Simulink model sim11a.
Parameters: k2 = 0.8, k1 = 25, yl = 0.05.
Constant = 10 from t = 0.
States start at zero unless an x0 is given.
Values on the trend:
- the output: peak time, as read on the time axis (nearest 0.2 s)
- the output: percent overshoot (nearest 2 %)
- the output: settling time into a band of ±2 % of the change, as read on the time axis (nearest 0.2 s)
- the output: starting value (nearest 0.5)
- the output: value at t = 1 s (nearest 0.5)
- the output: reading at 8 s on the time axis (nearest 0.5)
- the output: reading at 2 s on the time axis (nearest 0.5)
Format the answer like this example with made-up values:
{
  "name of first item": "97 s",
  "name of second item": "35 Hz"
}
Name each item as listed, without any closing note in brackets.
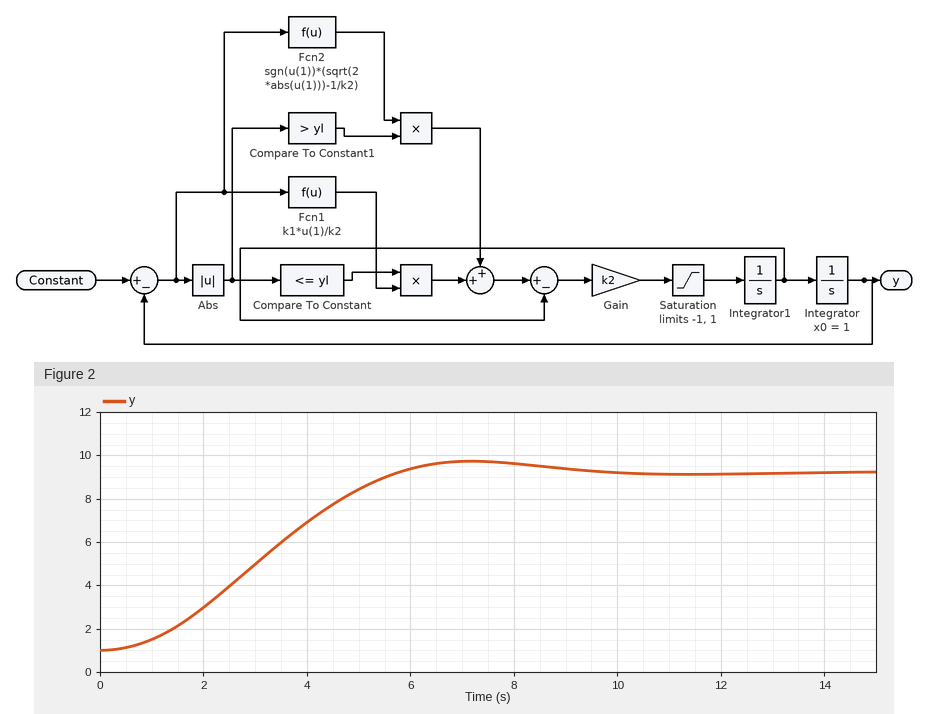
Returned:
{
  "the output: peak time, as read on the time axis": "7.2 s",
  "the output: percent overshoot": "6 %",
  "the output: settling time into a band of ±2 % of the change, as read on the time axis": "9.0 s",
  "the output: starting value": "1.0",
  "the output: value at t = 1 s": "1.5",
  "the output: reading at 8 s on the time axis": "9.5",
  "the output: reading at 2 s on the time axis": "3.0"
}
